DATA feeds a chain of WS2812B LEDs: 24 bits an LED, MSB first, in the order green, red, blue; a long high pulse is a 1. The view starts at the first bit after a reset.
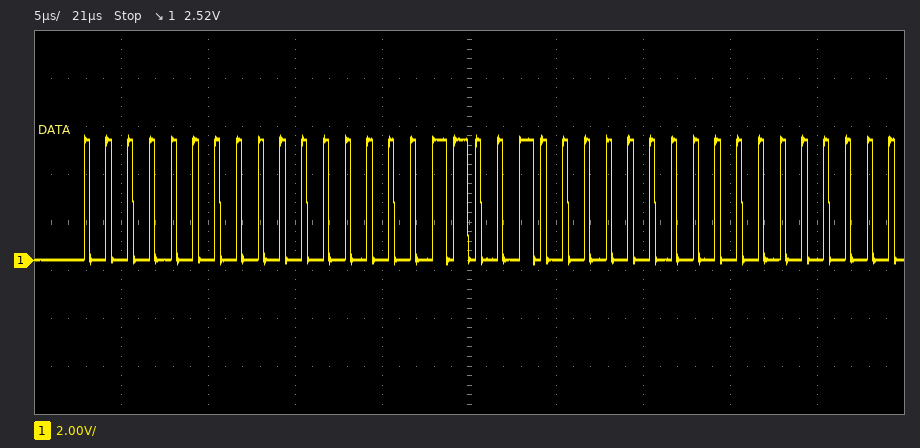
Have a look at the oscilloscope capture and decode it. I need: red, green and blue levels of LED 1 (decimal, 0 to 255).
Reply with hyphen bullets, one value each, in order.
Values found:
- 0, 0, 200
